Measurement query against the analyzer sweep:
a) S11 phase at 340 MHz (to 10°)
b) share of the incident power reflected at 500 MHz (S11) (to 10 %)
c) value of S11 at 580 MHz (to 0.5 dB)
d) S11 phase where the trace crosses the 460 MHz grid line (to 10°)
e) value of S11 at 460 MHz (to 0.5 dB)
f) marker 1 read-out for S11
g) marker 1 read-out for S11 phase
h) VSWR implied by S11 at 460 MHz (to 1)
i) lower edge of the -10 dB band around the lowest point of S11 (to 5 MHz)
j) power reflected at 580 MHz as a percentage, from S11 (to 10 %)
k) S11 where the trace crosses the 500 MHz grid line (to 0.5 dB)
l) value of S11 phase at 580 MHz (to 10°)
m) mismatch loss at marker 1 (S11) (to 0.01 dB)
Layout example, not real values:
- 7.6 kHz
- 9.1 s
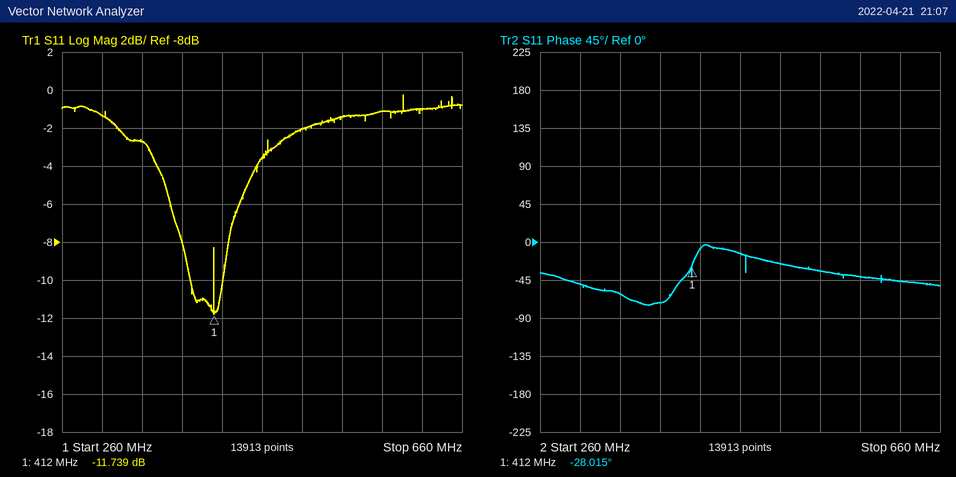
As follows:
- -60°
- 60 %
- -1.0 dB
- -10°
- -3.5 dB
- -11.739 dB
- -28.015°
- 5
- 390 MHz
- 80 %
- -2.0 dB
- -40°
- 0.30 dB
